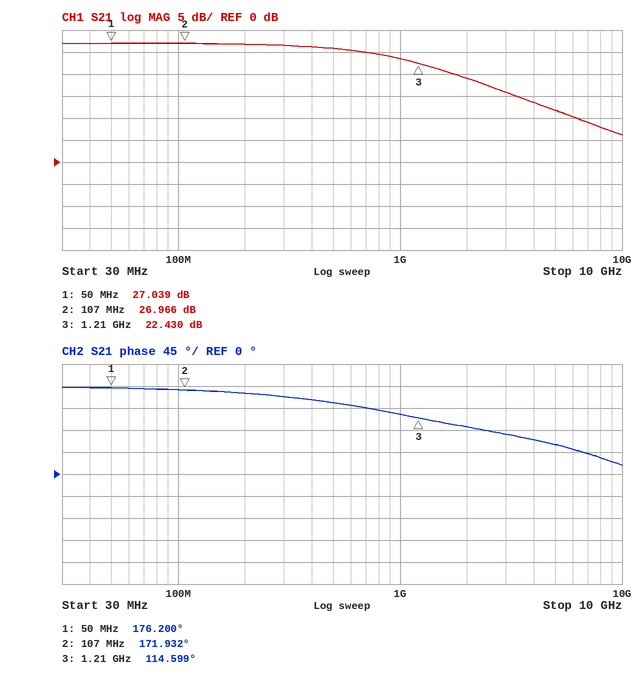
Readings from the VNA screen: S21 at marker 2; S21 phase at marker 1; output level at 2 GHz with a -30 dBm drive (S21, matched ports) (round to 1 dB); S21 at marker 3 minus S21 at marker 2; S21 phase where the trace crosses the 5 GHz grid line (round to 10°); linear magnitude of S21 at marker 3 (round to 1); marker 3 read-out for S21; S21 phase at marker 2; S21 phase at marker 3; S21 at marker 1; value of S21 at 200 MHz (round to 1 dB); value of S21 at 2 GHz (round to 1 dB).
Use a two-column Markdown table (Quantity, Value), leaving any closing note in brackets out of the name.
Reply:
| Quantity | Value |
|---|---|
| S21 at marker 2 | 26.966 dB |
| S21 phase at marker 1 | 176.200° |
| output level at 2 GHz with a -30 dBm drive (S21, matched ports) | -11 dBm |
| S21 at marker 3 minus S21 at marker 2 | -4.536 dB |
| S21 phase where the trace crosses the 5 GHz grid line | 60° |
| linear magnitude of S21 at marker 3 | 13 |
| marker 3 read-out for S21 | 22.430 dB |
| S21 phase at marker 2 | 171.932° |
| S21 phase at marker 3 | 114.599° |
| S21 at marker 1 | 27.039 dB |
| value of S21 at 200 MHz | 27 dB |
| value of S21 at 2 GHz | 19 dB |
